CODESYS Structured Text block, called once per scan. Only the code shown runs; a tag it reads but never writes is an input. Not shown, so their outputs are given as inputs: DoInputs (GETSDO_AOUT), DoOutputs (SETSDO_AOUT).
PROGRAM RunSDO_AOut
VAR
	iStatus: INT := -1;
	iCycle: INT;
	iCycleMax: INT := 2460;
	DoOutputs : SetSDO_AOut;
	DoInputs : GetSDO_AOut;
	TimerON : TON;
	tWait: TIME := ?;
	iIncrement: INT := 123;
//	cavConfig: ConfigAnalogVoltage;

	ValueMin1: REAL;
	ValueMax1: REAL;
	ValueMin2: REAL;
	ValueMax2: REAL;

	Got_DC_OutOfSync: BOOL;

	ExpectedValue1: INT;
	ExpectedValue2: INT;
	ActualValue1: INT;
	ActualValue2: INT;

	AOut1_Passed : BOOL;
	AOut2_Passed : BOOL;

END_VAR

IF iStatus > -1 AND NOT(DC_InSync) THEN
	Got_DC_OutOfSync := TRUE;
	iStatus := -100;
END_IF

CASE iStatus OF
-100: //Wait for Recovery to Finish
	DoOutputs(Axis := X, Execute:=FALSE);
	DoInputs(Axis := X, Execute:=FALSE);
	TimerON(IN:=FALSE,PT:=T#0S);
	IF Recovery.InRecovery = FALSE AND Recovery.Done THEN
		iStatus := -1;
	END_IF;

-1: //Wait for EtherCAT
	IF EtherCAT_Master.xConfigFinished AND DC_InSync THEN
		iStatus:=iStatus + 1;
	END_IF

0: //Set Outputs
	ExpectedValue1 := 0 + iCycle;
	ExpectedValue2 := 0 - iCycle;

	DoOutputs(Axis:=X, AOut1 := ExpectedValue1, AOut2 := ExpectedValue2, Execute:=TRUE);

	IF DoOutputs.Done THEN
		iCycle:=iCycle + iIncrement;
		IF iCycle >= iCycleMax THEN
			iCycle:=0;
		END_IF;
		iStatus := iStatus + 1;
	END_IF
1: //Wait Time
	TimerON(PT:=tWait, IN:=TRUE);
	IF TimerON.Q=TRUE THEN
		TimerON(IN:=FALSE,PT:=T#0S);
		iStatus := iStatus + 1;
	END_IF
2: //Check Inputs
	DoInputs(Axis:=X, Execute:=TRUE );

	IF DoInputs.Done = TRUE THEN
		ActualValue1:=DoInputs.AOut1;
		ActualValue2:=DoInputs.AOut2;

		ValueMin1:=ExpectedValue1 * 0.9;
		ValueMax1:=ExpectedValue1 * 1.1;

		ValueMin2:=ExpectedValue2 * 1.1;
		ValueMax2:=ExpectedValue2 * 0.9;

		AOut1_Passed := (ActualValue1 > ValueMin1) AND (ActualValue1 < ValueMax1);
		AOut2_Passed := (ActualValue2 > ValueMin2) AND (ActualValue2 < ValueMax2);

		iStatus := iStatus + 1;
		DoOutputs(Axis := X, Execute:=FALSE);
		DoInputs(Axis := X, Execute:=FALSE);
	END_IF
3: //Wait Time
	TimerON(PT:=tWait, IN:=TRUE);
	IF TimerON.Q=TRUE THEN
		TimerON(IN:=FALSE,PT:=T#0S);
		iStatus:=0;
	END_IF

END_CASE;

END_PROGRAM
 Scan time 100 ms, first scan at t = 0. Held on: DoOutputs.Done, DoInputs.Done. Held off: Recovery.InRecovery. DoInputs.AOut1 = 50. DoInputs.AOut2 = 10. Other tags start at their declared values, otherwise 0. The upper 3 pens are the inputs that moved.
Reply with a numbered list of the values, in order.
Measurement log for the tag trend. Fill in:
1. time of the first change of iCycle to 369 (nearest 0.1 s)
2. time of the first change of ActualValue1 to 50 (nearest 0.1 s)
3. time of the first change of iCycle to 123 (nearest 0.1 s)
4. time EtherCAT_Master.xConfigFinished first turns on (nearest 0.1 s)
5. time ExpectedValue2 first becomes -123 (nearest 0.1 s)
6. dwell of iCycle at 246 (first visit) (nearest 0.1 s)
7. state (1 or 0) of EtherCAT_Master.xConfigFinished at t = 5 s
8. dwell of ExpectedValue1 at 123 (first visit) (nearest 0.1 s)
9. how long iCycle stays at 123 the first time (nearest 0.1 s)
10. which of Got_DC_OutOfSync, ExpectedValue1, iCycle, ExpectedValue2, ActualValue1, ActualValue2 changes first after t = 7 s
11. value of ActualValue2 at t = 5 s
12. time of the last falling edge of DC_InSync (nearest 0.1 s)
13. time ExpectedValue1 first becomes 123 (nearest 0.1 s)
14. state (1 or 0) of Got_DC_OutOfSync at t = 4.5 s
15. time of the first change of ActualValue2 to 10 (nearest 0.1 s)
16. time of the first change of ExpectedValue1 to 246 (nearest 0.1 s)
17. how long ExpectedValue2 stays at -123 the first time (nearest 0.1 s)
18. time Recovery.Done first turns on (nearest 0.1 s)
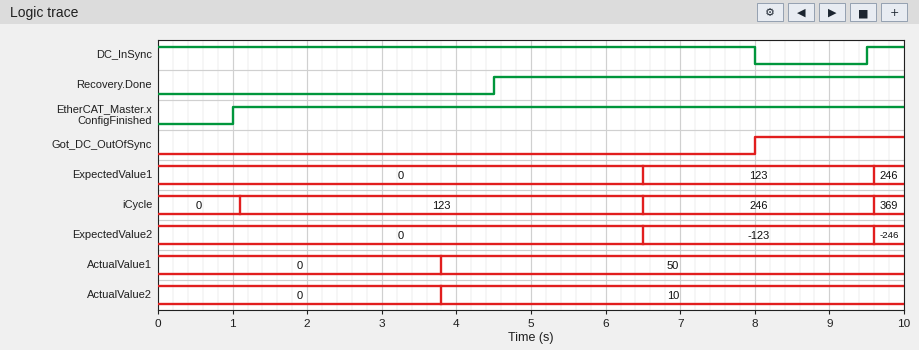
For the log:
1. 9.6 s
2. 3.8 s
3. 1.1 s
4. 1.0 s
5. 6.5 s
6. 3.1 s
7. 1
8. 3.1 s
9. 5.4 s
10. Got_DC_OutOfSync
11. 10
12. 8.0 s
13. 6.5 s
14. 0
15. 3.8 s
16. 9.6 s
17. 3.1 s
18. 4.5 s
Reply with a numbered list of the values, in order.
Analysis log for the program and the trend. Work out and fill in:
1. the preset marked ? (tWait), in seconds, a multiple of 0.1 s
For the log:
1. 2.5 s
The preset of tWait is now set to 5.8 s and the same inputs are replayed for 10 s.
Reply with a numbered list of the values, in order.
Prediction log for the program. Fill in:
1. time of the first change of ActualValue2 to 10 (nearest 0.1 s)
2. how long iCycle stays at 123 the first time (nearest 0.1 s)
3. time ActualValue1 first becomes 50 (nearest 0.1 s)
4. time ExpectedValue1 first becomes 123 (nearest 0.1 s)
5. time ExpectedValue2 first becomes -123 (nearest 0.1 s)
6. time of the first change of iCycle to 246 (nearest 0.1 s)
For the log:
1. 7.1 s
2. 8.5 s
3. 7.1 s
4. 9.6 s
5. 9.6 s
6. 9.6 s
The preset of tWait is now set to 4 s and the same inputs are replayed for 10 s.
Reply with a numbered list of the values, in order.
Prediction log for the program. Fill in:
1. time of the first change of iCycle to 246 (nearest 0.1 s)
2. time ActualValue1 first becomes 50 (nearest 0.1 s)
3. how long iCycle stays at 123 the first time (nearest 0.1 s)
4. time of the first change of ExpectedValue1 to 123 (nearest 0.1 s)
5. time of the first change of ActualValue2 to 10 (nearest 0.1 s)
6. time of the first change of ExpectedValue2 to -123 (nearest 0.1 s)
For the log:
1. 9.6 s
2. 5.3 s
3. 8.5 s
4. 9.6 s
5. 5.3 s
6. 9.6 s
